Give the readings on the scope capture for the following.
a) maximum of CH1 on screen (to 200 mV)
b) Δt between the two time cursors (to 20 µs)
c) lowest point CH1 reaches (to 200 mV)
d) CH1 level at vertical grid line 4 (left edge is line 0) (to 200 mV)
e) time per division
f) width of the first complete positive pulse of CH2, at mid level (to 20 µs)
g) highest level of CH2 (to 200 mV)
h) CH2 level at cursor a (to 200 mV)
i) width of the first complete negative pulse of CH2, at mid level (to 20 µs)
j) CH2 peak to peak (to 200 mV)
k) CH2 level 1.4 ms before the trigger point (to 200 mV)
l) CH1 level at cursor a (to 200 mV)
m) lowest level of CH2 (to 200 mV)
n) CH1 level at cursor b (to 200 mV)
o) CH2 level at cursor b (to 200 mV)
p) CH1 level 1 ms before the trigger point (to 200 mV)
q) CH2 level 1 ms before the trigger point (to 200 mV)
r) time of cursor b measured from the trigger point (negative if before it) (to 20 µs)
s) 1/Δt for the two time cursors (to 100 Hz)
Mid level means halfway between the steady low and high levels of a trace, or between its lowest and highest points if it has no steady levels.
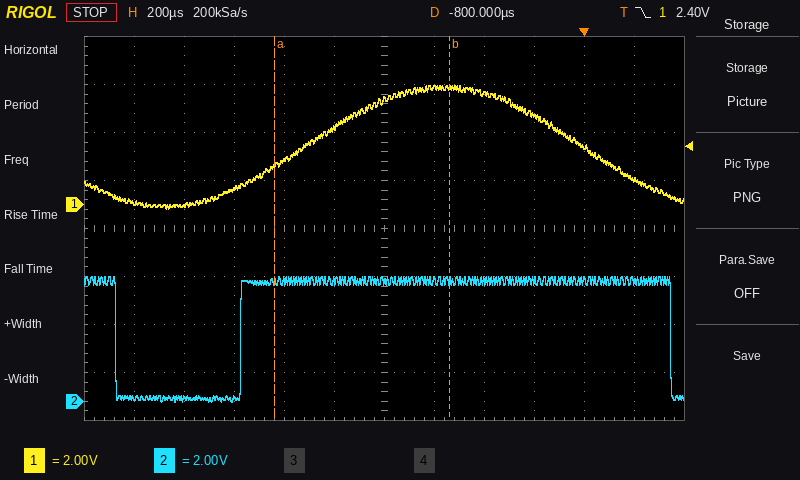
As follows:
5.0 V
700 µs
-200 mV
1.8 V
200 µs
1.72 ms
5.2 V
5.0 V
500 µs
5.2 V
200 mV
1.6 V
0.0 V
4.8 V
5.0 V
3.2 V
5.0 V
-540 µs
1.4 kHz
